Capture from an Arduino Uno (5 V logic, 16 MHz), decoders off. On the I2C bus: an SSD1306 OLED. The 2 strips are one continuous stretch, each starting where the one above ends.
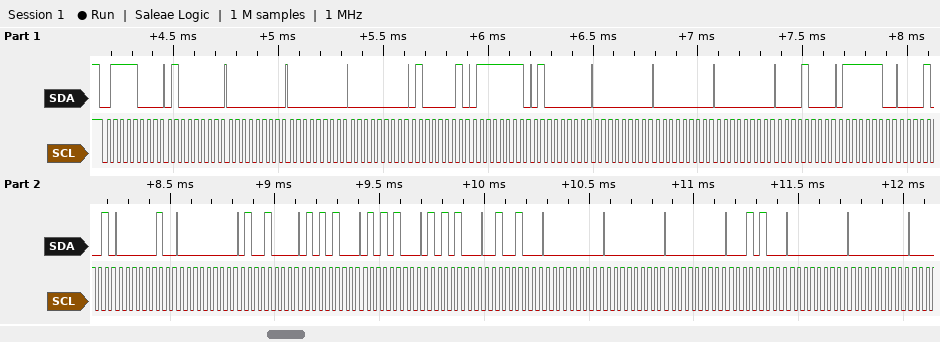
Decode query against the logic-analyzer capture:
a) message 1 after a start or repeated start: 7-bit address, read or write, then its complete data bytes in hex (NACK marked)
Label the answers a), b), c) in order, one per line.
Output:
a) 0x3C write: 40 00 00 00 41 7F 40 00 00 00 08 7E 09 02 00 48 54 54 54 24 00 00 00 14 00 00
